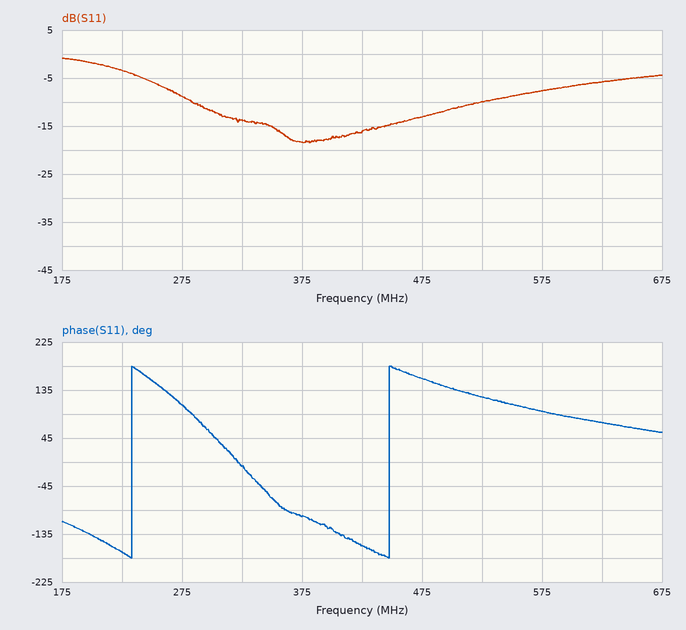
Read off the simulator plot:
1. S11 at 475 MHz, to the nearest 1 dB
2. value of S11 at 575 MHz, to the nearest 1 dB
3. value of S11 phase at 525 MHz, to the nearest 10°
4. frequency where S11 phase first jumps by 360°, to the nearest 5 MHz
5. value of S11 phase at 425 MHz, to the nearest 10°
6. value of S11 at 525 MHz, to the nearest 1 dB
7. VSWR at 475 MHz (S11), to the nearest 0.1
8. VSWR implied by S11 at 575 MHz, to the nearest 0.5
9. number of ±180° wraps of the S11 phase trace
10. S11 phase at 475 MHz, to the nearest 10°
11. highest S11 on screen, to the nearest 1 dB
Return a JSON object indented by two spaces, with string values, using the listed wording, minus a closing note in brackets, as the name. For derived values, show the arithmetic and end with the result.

{
  "S11 at 475 MHz, to the nearest 1 dB": "-13 dB",
  "value of S11 at 575 MHz, to the nearest 1 dB": "-8 dB",
  "value of S11 phase at 525 MHz, to the nearest 10°": "120°",
  "frequency where S11 phase first jumps by 360°, to the nearest 5 MHz": "235 MHz",
  "value of S11 phase at 425 MHz, to the nearest 10°": "-160°",
  "value of S11 at 525 MHz, to the nearest 1 dB": "-10 dB",
  "VSWR at 475 MHz (S11), to the nearest 0.1": "|Γ| = 10^(-13/20) = 0.2239; VSWR = (1 + 0.2239)/(1 − 0.2239) ≈ 1.6",
  "VSWR implied by S11 at 575 MHz, to the nearest 0.5": "|Γ| = 10^(-8/20) = 0.3981; VSWR = (1 + 0.3981)/(1 − 0.3981) ≈ 2.32, so 2.5 to the nearest 0.5",
  "number of ±180° wraps of the S11 phase trace": "2",
  "S11 phase at 475 MHz, to the nearest 10°": "160°",
  "highest S11 on screen, to the nearest 1 dB": "-1 dB"
}
